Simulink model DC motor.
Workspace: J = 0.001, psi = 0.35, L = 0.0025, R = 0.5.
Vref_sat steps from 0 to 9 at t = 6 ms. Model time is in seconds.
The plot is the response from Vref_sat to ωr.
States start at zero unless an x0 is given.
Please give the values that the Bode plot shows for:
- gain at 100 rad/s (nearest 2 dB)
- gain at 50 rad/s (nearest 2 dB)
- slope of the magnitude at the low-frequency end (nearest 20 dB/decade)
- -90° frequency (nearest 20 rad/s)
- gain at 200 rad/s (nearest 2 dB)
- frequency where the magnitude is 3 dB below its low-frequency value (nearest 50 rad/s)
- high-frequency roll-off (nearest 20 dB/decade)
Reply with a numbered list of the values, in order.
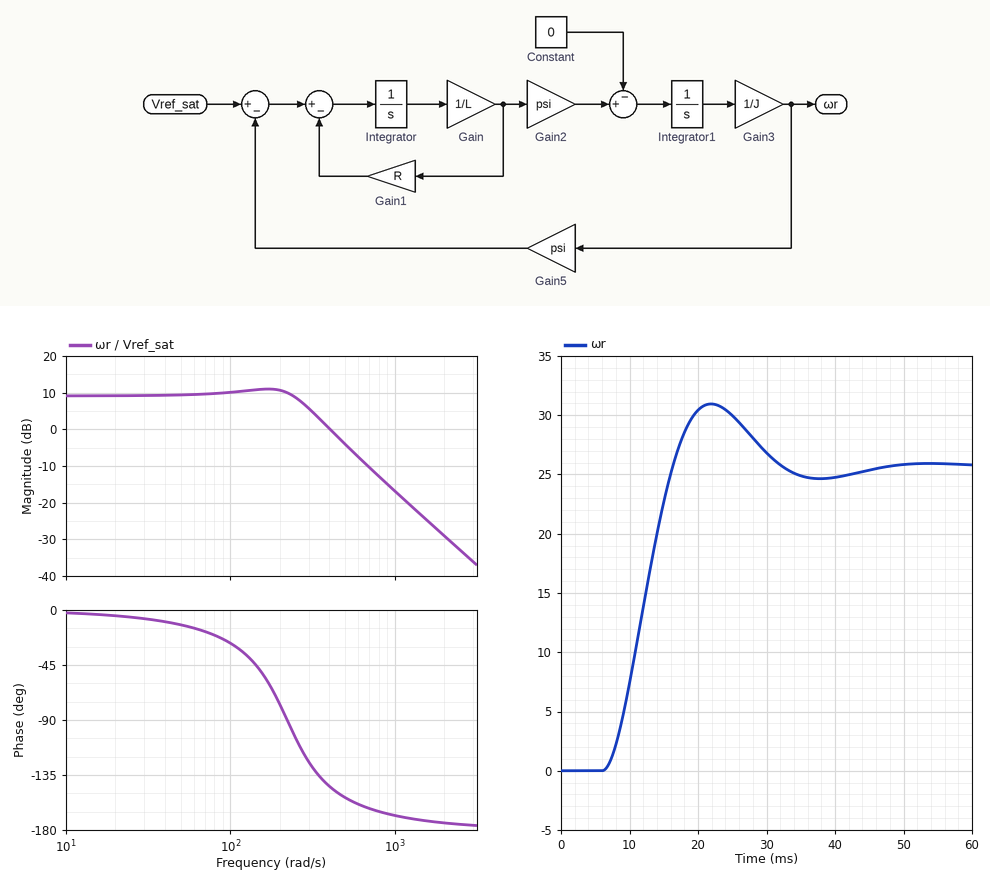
1. 10 dB
2. 10 dB
3. 0 dB/decade
4. 220 rad/s
5. 10 dB
6. 300 rad/s
7. -40 dB/decade
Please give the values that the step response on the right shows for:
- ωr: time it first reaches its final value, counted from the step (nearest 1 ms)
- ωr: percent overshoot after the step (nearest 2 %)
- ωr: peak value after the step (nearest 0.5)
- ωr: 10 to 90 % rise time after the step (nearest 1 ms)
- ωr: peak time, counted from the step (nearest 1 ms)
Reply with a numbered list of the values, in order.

1. 10 ms
2. 20 %
3. 31.0
4. 7 ms
5. 16 ms
